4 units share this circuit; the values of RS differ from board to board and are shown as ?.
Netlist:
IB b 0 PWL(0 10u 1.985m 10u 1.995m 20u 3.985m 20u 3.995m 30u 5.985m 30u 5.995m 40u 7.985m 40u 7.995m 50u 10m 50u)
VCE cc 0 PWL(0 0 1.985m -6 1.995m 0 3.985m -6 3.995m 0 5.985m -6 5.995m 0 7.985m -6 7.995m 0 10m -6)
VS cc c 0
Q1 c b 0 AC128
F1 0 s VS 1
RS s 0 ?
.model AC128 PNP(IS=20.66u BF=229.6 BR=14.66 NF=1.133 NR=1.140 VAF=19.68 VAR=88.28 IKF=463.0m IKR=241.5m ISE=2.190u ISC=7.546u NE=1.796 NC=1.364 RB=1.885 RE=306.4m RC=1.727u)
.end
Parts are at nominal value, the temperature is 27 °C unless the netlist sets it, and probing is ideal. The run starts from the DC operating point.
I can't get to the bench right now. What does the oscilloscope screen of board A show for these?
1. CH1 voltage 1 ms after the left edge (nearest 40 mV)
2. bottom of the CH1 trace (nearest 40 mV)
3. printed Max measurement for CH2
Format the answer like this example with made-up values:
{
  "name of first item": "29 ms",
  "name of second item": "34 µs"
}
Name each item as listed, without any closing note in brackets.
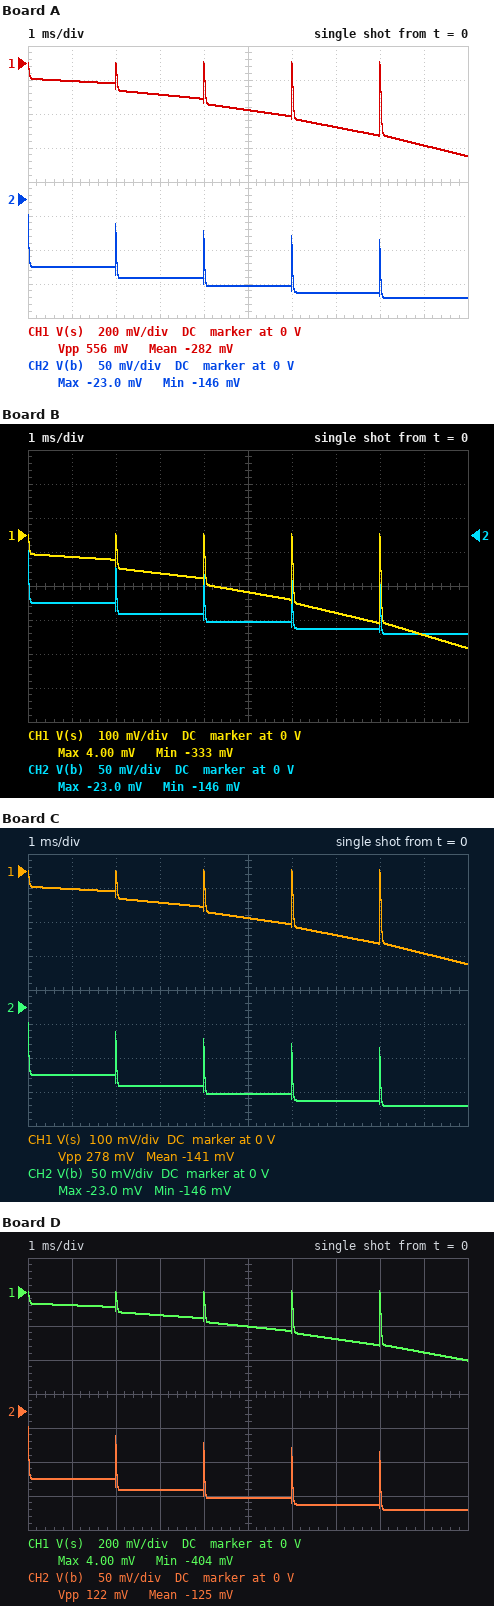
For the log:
{
  "CH1 voltage 1 ms after the left edge": "-120 mV",
  "bottom of the CH1 trace": "-560 mV",
  "printed Max measurement for CH2": "-23.0 mV"
}
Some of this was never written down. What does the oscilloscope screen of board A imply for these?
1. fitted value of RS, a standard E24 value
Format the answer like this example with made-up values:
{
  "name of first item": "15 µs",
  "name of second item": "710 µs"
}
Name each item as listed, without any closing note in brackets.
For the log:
{
  "fitted value of RS, a standard E24 value": "150 Ω"
}
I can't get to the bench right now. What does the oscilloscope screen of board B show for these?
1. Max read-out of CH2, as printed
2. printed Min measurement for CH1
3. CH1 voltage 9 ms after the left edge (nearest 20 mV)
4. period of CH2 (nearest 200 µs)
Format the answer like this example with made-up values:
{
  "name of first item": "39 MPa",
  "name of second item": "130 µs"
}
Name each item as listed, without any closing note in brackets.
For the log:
{
  "Max read-out of CH2, as printed": "-23.0 mV",
  "printed Min measurement for CH1": "-333 mV",
  "CH1 voltage 9 ms after the left edge": "-300 mV",
  "period of CH2": "2.0 ms"
}
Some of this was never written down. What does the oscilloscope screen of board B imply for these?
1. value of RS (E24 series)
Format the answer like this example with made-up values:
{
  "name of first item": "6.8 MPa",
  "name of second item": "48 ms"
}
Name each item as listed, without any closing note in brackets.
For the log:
{
  "value of RS": "91 Ω"
}
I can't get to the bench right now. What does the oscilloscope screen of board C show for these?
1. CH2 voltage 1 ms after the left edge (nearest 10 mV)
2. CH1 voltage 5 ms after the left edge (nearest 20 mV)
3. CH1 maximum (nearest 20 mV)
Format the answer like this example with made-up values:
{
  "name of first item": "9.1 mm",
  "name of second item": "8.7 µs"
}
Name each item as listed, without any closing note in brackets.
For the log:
{
  "CH2 voltage 1 ms after the left edge": "-100 mV",
  "CH1 voltage 5 ms after the left edge": "-140 mV",
  "CH1 maximum": "0 V"
}
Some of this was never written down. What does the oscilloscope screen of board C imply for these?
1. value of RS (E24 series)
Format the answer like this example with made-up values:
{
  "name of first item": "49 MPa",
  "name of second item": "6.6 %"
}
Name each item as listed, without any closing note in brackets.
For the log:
{
  "value of RS": "75 Ω"
}
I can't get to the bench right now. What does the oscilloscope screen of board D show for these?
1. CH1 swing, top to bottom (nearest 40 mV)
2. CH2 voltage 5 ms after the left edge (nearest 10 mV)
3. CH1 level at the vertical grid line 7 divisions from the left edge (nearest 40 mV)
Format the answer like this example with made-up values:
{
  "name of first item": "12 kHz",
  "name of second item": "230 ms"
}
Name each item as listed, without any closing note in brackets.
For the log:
{
  "CH1 swing, top to bottom": "400 mV",
  "CH2 voltage 5 ms after the left edge": "-130 mV",
  "CH1 level at the vertical grid line 7 divisions from the left edge": "-280 mV"
}
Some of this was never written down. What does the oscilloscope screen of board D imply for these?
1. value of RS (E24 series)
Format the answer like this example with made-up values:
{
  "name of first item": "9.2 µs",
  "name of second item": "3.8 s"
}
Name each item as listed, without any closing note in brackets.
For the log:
{
  "value of RS": "110 Ω"
}
